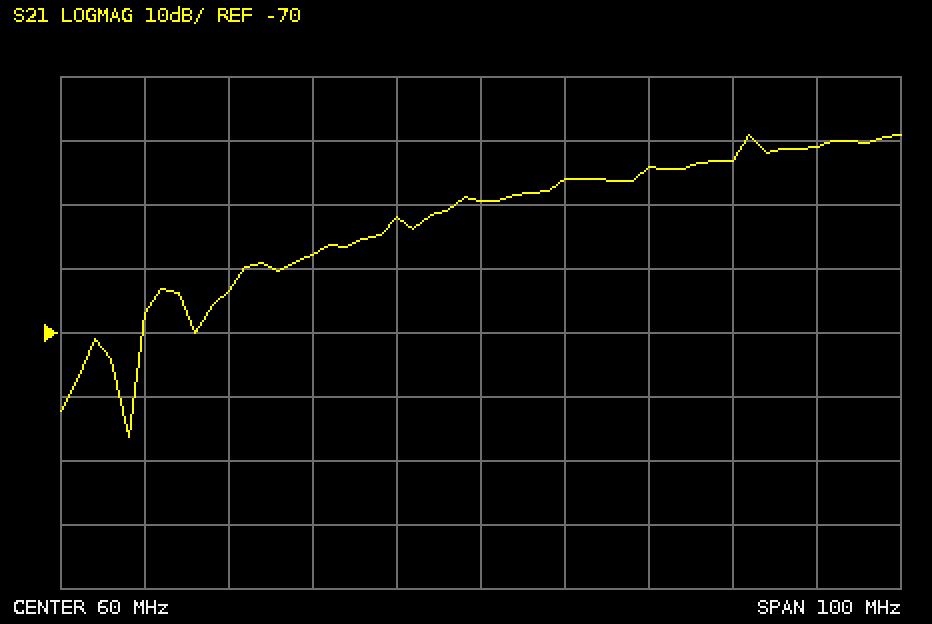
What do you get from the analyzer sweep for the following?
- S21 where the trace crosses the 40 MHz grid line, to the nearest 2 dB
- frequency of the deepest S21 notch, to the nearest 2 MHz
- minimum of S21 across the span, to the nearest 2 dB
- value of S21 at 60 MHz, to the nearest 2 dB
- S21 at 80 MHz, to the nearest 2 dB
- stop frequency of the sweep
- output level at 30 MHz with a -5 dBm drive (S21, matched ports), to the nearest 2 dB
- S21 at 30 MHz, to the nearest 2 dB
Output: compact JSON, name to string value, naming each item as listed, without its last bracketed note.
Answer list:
{"S21 where the trace crosses the 40 MHz grid line, to the nearest 2 dB": "-58 dB", "frequency of the deepest S21 notch, to the nearest 2 MHz": "18 MHz", "minimum of S21 across the span, to the nearest 2 dB": "-86 dB", "value of S21 at 60 MHz, to the nearest 2 dB": "-50 dB", "S21 at 80 MHz, to the nearest 2 dB": "-44 dB", "stop frequency of the sweep": "110 MHz", "output level at 30 MHz with a -5 dBm drive (S21, matched ports), to the nearest 2 dB": "-68 dBm", "S21 at 30 MHz, to the nearest 2 dB": "-64 dB"}
